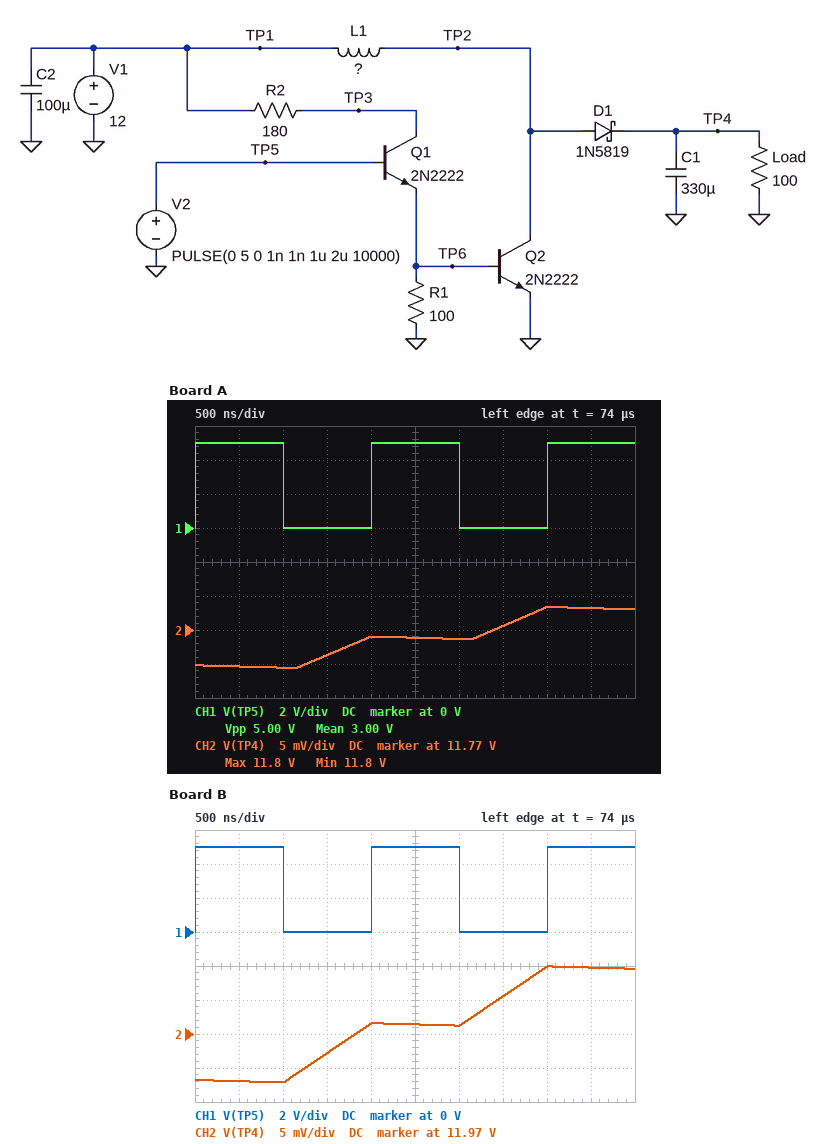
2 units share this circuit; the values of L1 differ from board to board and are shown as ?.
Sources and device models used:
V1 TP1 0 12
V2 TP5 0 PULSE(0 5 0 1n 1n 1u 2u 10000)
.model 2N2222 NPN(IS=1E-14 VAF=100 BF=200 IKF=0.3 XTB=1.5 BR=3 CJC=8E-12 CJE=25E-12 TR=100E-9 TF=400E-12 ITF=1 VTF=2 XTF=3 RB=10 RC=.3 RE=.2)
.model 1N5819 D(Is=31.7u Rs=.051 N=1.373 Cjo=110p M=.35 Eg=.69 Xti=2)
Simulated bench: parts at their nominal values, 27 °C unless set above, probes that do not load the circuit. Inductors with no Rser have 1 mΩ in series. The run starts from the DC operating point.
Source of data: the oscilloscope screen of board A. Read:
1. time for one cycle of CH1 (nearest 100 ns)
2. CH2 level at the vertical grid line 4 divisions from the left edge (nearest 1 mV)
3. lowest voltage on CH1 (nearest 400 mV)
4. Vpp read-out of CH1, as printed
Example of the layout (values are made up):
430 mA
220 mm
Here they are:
2.0 µs
11.764 V
0 V
5.00 V
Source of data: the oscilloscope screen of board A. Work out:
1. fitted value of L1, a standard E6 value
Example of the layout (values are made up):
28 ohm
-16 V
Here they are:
330 µH
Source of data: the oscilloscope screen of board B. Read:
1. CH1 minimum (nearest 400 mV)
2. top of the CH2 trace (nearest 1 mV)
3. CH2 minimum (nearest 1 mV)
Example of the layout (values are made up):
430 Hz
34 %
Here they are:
0 V
11.985 V
11.968 V
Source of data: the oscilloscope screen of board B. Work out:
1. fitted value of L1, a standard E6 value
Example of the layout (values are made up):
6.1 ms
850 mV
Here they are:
47 µH
